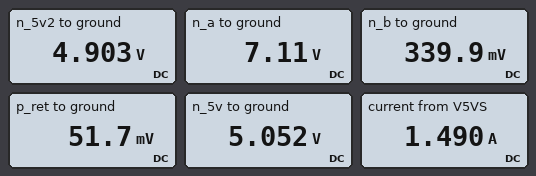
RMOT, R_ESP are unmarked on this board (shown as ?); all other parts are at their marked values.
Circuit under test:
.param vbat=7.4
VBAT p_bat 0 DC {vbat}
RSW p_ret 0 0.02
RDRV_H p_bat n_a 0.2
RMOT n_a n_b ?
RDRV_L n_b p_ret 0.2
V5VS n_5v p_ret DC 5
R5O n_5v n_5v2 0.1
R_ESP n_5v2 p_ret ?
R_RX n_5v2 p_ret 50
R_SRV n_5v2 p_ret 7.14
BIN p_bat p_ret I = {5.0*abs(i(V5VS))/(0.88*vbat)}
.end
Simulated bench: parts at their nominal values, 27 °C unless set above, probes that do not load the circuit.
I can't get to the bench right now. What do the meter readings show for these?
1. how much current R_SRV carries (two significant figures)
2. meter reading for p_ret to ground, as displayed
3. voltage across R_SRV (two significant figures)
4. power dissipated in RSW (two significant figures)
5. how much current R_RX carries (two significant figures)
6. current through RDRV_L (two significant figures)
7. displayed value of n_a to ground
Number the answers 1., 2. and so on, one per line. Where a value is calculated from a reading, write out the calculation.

1. (4.903 V - 51.7 mV) / 7.14 Ω = 680 mA
2. 51.7 mV
3. 4.903 V - 51.7 mV = 4.9 V
4. (51.7 mV)^2 / 20 mΩ = 130 mW
5. (4.903 V - 51.7 mV) / 50 Ω = 97 mA
6. (339.9 mV - 51.7 mV) / 200 mΩ = 1.4 A
7. 7.11 V
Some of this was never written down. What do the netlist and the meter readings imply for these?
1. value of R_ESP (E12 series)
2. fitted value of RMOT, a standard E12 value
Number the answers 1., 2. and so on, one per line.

1. 6.8 Ω
2. 4.7 Ω
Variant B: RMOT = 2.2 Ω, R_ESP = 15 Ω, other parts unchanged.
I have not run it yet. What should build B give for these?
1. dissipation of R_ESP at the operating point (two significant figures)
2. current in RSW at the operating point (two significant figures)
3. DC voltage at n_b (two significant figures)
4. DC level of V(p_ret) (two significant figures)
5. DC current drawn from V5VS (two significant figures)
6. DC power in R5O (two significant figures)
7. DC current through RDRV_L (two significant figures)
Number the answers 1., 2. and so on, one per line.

1. 1.6 W
2. 3.7 A
3. 640 mV
4. 73 mV
5. 1.1 A
6. 120 mW
7. 2.8 A
